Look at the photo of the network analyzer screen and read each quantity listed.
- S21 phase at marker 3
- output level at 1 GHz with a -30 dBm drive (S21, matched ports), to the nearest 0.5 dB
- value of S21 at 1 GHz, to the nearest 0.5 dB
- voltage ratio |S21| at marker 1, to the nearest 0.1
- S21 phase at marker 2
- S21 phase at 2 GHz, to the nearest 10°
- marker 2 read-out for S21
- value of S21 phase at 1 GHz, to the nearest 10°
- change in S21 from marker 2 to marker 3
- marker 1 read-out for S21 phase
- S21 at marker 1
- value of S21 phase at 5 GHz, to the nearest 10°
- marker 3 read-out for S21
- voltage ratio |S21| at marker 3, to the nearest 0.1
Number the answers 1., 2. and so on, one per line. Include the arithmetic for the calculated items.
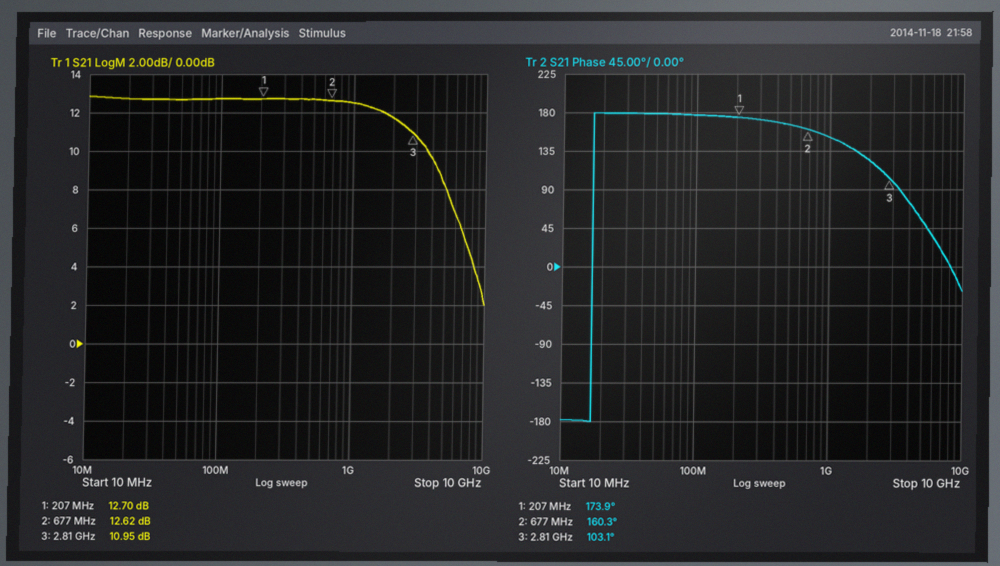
1. 103.1°
2. -30 dBm + (12.5 dB) = -17.5 dBm
3. 12.5 dB
4. 10^(12.7/20) ≈ 4.3
5. 160.3°
6. 120°
7. 12.62 dB
8. 150°
9. 10.95 − (12.62) = -1.67 dB
10. 173.9°
11. 12.70 dB
12. 50°
13. 10.95 dB
14. 10^(10.95/20) ≈ 3.5
